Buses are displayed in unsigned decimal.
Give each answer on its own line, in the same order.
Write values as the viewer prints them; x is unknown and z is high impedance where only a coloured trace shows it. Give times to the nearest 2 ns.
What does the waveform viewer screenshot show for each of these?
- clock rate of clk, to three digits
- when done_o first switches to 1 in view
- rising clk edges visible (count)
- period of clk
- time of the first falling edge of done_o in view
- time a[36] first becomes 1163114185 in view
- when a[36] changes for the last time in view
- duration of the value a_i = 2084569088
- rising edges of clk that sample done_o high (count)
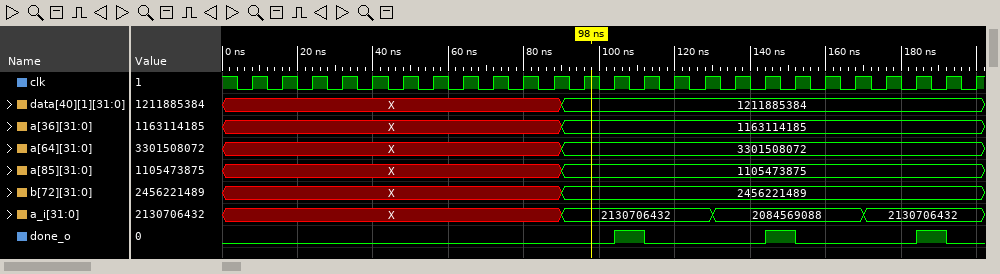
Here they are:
125 MHz
104 ns
25
8 ns
112 ns
90 ns
90 ns
40 ns
3
